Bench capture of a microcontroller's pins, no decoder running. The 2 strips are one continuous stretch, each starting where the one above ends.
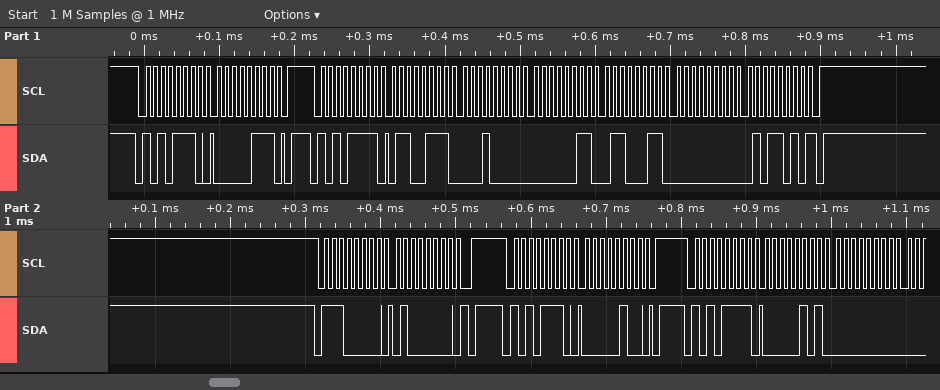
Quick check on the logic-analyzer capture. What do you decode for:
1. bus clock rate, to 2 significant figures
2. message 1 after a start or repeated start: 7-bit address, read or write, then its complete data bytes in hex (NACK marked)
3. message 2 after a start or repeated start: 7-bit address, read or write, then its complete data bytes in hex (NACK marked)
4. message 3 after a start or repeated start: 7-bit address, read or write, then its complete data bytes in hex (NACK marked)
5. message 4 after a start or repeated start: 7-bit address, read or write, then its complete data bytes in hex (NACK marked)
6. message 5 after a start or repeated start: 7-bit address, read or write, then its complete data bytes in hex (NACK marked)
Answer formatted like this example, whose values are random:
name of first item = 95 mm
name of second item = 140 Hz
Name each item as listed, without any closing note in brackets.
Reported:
bus clock rate, to 2 significant figures = 100 kHz
message 1 after a start or repeated start: 7-bit address, read or write, then its complete data bytes in hex = 0x57 write: 07
message 2 after a start or repeated start: 7-bit address, read or write, then its complete data bytes in hex = 0x57 read: 67 10 03 63 00 5A NACK
message 3 after a start or repeated start: 7-bit address, read or write, then its complete data bytes in hex = 0x70 write: 40
message 4 after a start or repeated start: 7-bit address, read or write, then its complete data bytes in hex = 0x57 write: 04
message 5 after a start or repeated start: 7-bit address, read or write, then its complete data bytes in hex = 0x57 read: 05 00
